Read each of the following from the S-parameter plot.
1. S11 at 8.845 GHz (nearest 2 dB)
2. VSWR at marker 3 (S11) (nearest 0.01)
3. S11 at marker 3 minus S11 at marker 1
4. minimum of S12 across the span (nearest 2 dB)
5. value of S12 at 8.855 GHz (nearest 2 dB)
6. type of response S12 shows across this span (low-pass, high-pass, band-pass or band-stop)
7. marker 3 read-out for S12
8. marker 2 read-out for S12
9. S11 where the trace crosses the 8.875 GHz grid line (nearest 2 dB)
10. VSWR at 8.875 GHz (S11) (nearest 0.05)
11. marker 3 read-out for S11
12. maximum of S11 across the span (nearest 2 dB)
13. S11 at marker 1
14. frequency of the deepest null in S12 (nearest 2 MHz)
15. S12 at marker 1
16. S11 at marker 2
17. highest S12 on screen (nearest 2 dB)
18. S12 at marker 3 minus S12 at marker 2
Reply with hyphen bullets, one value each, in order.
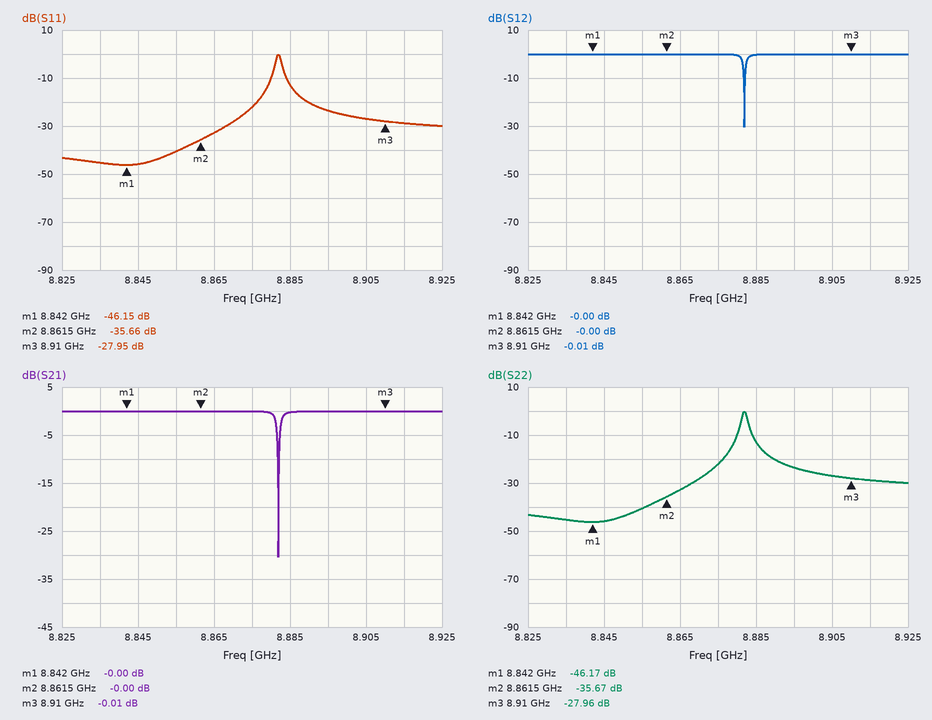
- -46 dB
- 1.08
- 18.20 dB
- -30 dB
- 0 dB
- band-stop
- -0.01 dB
- -0.00 dB
- -22 dB
- 1.15
- -27.95 dB
- 0 dB
- -46.15 dB
- 8.882 GHz
- -0.00 dB
- -35.66 dB
- 0 dB
- -0.01 dB
